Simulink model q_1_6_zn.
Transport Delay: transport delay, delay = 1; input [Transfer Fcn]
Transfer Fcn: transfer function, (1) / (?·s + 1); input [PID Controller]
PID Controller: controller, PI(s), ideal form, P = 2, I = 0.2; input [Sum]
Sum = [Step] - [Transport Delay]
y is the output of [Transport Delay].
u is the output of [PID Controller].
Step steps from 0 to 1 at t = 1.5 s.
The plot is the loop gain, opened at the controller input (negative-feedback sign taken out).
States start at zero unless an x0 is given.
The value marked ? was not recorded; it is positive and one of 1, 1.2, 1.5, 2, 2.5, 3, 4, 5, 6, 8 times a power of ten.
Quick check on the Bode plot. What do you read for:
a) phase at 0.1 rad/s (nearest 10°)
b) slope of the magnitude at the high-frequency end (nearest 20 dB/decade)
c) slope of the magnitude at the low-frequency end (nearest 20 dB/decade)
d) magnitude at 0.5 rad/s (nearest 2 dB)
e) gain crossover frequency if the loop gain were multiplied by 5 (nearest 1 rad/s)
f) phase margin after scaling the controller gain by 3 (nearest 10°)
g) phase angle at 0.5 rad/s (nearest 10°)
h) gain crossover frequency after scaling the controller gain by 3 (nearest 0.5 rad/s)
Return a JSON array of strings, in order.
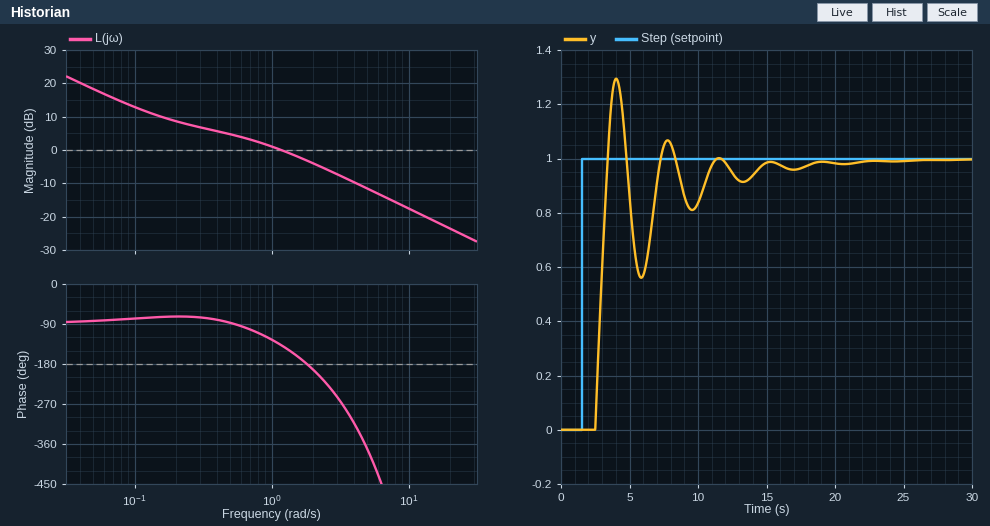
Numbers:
["-80°", "-20 dB/decade", "-20 dB/decade", "4 dB", "7 rad/s", "-130°", "-90°", "4.0 rad/s"]
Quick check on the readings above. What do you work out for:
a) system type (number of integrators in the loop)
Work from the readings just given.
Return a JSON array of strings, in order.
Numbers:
["1"]
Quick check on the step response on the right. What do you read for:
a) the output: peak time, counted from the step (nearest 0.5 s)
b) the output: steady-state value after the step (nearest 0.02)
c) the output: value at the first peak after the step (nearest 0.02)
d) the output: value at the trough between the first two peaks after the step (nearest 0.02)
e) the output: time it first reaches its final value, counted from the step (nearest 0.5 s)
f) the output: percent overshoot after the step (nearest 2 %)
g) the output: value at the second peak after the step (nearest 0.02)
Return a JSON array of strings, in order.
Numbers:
["2.5 s", "1.00", "1.30", "0.56", "2.0 s", "30 %", "1.06"]
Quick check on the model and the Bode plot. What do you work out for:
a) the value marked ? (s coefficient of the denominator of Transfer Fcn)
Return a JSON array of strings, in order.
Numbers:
["1.5"]
